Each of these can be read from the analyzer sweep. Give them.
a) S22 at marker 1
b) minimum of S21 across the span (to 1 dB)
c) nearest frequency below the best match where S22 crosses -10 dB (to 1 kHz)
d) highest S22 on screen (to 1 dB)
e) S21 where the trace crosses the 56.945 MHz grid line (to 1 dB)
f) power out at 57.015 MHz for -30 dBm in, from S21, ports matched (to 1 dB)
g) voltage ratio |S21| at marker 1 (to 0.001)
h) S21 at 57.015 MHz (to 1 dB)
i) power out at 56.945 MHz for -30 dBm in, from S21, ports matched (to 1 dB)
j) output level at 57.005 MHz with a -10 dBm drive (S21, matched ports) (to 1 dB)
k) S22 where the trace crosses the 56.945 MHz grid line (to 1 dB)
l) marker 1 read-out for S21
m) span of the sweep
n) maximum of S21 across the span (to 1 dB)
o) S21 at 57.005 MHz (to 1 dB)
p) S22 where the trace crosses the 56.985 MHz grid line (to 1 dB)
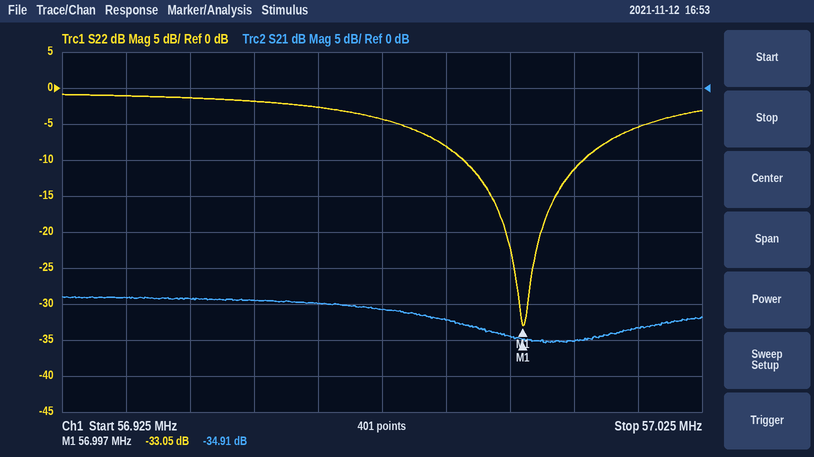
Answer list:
-33.05 dB
-35 dB
56.988 MHz
-1 dB
-29 dB
-63 dBm
0.018
-33 dB
-59 dBm
-45 dBm
-1 dB
-34.91 dB
100 kHz
-29 dB
-35 dB
-8 dB
